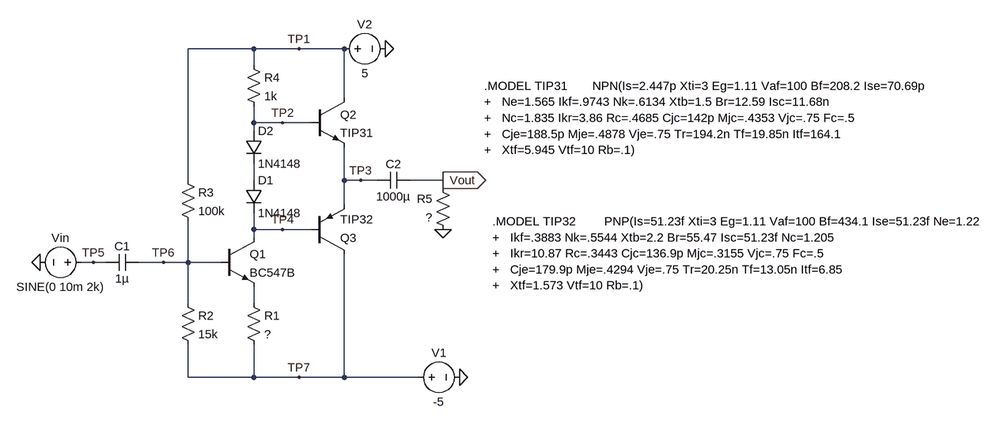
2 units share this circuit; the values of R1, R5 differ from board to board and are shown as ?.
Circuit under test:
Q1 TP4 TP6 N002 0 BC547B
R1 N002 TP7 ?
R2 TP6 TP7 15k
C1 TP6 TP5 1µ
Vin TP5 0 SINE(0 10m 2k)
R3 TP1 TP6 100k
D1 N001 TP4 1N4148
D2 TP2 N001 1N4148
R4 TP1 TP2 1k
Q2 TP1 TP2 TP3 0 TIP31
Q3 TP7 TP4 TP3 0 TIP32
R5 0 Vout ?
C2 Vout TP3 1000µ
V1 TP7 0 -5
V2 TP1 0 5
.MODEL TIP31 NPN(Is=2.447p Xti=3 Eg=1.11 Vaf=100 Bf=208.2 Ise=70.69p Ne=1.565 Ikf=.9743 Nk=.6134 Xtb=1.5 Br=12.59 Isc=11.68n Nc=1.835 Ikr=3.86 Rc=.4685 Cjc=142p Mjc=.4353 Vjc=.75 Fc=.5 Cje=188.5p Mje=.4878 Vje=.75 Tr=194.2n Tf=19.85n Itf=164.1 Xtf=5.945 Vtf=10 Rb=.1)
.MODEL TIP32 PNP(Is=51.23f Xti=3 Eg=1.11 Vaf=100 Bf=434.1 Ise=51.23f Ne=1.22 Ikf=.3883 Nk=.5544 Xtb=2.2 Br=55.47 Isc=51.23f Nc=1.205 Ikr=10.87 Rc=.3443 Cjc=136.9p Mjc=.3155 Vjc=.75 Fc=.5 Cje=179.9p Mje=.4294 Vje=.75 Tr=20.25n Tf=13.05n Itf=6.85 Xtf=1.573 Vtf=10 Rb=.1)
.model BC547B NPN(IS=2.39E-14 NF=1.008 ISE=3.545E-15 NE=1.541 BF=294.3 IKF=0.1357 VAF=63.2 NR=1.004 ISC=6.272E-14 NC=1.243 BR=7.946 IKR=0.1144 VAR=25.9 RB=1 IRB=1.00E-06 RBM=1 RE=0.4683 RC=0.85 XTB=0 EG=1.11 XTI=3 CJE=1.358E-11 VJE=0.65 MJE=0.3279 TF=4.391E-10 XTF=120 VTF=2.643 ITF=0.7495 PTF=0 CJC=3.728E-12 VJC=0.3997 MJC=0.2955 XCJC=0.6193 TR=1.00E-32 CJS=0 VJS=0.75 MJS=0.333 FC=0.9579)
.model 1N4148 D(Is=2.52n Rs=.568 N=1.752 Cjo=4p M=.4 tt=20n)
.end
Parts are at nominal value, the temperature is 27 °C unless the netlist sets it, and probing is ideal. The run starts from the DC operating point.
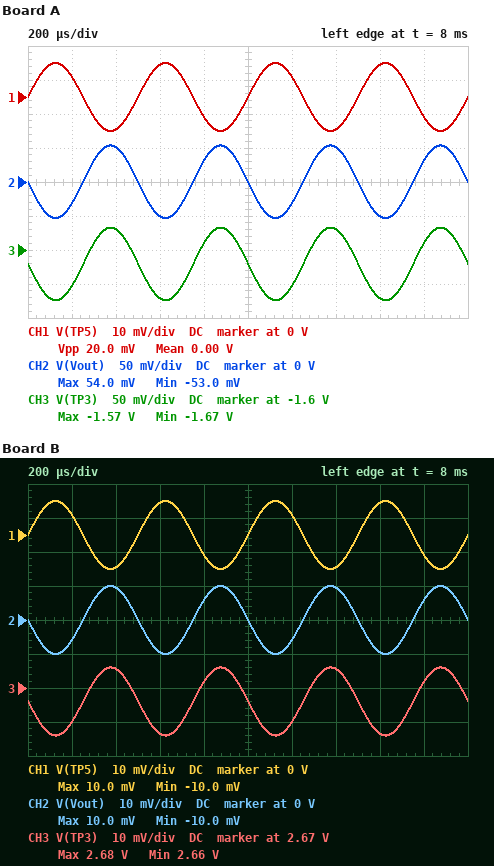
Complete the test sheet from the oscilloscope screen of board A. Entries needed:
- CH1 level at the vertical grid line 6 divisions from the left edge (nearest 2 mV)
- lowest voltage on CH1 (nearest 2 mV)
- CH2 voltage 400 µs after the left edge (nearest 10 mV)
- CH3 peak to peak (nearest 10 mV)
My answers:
6 mV
-10 mV
50 mV
110 mV
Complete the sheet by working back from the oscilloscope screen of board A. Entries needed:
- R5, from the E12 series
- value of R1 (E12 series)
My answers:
4.7 Ω
56 Ω
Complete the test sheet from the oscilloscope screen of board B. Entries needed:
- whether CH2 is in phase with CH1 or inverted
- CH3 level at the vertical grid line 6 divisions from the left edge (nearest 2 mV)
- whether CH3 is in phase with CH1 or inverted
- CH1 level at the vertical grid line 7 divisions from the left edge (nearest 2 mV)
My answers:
inverted
2.660 V
inverted
-10 mV
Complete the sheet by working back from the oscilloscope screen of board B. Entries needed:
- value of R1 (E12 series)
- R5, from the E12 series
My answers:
330 Ω
6.8 Ω
